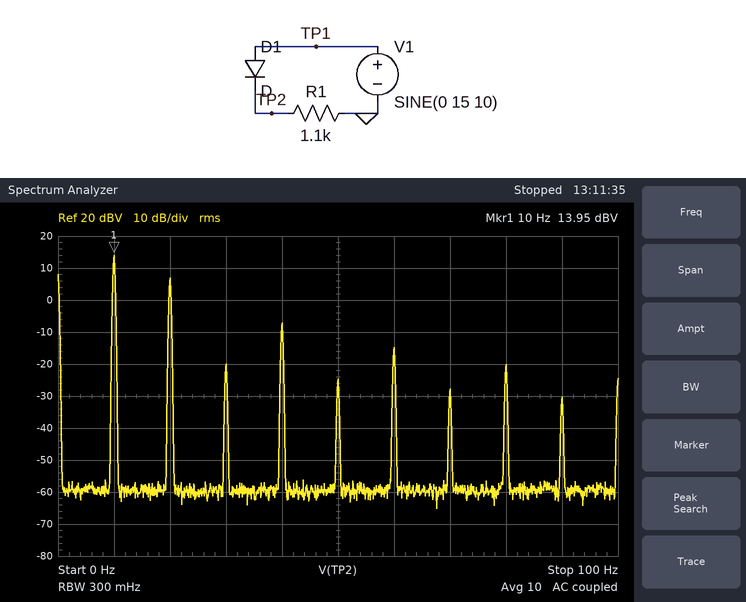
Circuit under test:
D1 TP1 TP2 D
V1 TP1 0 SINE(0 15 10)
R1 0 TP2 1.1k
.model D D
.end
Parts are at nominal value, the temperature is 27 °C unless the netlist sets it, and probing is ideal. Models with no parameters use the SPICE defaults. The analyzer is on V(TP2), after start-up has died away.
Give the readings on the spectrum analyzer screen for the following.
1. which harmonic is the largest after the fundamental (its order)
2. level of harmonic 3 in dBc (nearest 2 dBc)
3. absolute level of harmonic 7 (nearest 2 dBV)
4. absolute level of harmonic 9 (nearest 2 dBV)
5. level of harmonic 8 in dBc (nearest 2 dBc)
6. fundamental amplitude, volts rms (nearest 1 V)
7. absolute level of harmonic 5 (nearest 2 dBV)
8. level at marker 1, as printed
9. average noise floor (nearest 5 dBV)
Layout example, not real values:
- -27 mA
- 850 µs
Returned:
- 2
- -34 dBc
- -28 dBV
- -30 dBV
- -34 dBc
- 5 V
- -24 dBV
- 13.95 dBV
- -60 dBV
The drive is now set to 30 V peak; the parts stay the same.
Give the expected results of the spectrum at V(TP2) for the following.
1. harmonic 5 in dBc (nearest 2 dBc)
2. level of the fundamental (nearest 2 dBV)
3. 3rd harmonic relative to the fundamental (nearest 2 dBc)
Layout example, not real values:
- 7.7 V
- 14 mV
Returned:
- -44 dBc
- 20 dBV
- -40 dBc
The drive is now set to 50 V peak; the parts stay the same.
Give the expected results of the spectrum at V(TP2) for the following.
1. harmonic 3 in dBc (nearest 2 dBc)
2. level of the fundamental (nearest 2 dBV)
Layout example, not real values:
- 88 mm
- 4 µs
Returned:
- -44 dBc
- 24 dBV
